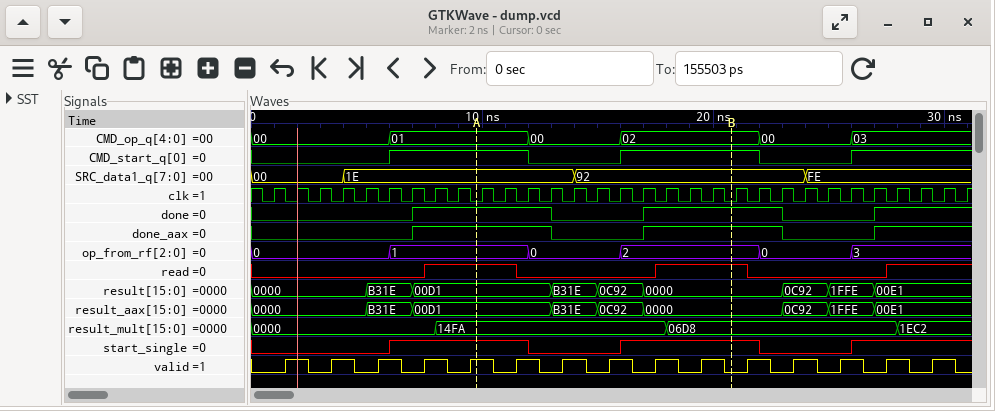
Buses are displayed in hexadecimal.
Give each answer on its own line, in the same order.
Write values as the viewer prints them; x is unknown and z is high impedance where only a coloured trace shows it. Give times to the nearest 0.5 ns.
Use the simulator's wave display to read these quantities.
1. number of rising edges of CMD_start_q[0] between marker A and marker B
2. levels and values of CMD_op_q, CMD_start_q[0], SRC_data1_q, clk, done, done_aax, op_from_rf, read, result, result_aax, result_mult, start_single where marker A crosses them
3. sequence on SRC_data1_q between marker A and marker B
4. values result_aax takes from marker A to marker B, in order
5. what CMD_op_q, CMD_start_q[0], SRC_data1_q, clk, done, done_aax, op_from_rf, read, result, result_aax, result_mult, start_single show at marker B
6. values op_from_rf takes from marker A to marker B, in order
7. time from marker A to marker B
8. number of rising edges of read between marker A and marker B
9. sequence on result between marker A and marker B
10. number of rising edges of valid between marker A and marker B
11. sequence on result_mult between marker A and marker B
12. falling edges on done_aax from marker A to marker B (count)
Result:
1
CMD_op_q=01, CMD_start_q[0]=1, SRC_data1_q=1E, clk=0, done=1, done_aax=1, op_from_rf=1, read=1, result=00D1, result_aax=00D1, result_mult=14FA, start_single=1
1E, 92
00D1, B31E, 0C92, 0000
CMD_op_q=02, CMD_start_q[0]=1, SRC_data1_q=92, clk=0, done=1, done_aax=1, op_from_rf=2, read=1, result=0000, result_aax=0000, result_mult=06D8, start_single=1
1, 0, 2
11 ns
1
00D1, B31E, 0C92, 0000
5
14FA, 06D8
1
